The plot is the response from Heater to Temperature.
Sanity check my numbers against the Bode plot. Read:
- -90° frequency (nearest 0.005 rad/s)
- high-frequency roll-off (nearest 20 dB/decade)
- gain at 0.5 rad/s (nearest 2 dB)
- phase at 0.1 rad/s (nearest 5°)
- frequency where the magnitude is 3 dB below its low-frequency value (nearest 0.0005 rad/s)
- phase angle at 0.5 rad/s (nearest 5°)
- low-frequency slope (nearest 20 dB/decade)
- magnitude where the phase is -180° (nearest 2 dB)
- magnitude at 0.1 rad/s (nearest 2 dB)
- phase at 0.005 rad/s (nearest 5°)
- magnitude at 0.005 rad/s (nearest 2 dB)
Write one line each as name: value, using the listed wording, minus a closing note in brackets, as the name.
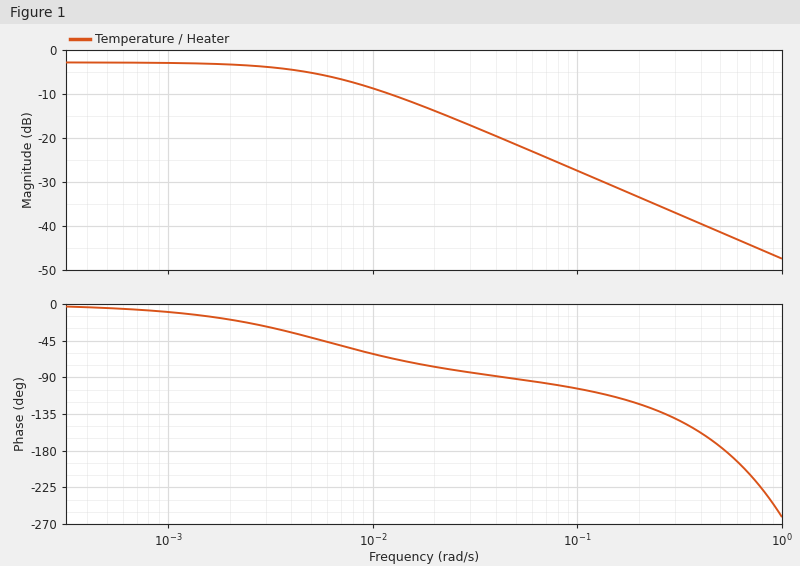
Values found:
-90° frequency: 0.045 rad/s
high-frequency roll-off: -20 dB/decade
gain at 0.5 rad/s: -42 dB
phase at 0.1 rad/s: -105°
frequency where the magnitude is 3 dB below its low-frequency value: 0.0060 rad/s
phase angle at 0.5 rad/s: -175°
low-frequency slope: 0 dB/decade
magnitude where the phase is -180°: -42 dB
magnitude at 0.1 rad/s: -28 dB
phase at 0.005 rad/s: -40°
magnitude at 0.005 rad/s: -6 dB
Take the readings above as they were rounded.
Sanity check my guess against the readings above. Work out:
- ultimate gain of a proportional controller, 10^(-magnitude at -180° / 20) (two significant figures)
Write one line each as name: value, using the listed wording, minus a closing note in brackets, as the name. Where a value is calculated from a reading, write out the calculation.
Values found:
ultimate gain of a proportional controller, 10^(-magnitude at -180° / 20): 10^(42 / 20) = 130
